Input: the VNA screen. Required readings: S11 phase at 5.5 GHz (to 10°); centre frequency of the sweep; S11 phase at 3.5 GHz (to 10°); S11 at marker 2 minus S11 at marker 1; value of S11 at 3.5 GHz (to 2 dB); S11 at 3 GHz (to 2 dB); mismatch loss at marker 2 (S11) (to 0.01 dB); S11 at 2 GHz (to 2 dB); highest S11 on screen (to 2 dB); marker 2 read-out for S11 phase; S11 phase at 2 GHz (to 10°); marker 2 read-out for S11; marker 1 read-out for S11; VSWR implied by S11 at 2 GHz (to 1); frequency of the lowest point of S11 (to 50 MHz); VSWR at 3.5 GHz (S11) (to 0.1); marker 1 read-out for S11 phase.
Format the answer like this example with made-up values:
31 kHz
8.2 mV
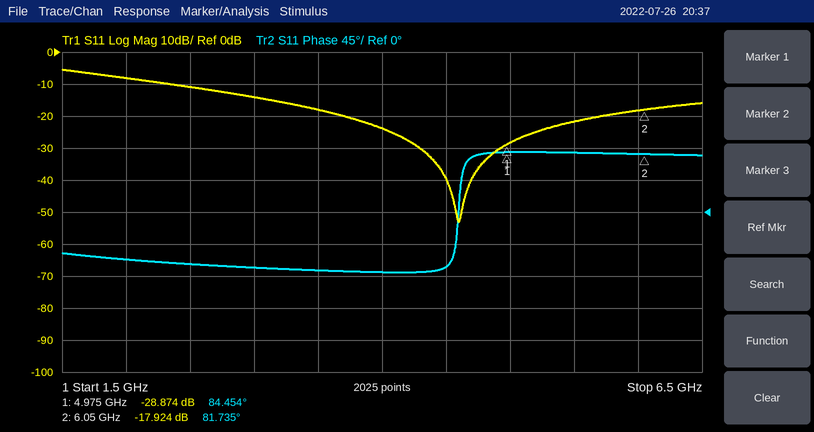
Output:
80°
4 GHz
-80°
10.950 dB
-18 dB
-14 dB
0.07 dB
-8 dB
-6 dB
81.735°
-70°
-17.924 dB
-28.874 dB
2
4.60 GHz
1.3
84.454°
